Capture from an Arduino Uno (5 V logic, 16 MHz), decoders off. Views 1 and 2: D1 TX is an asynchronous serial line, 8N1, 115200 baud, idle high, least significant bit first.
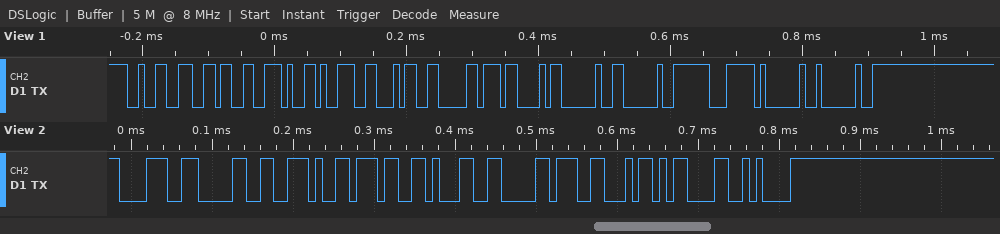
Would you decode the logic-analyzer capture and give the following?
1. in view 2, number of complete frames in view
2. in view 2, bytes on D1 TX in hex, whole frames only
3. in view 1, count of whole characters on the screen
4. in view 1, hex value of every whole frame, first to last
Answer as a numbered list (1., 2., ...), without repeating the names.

1. 9
2. 0x38 0x30 0x2E 0x37 0x31 0xB0 0x46 0x0D 0x0A
3. 12
4. 32 36 2E 39 34 B0 43 20 20 7C 20 20
